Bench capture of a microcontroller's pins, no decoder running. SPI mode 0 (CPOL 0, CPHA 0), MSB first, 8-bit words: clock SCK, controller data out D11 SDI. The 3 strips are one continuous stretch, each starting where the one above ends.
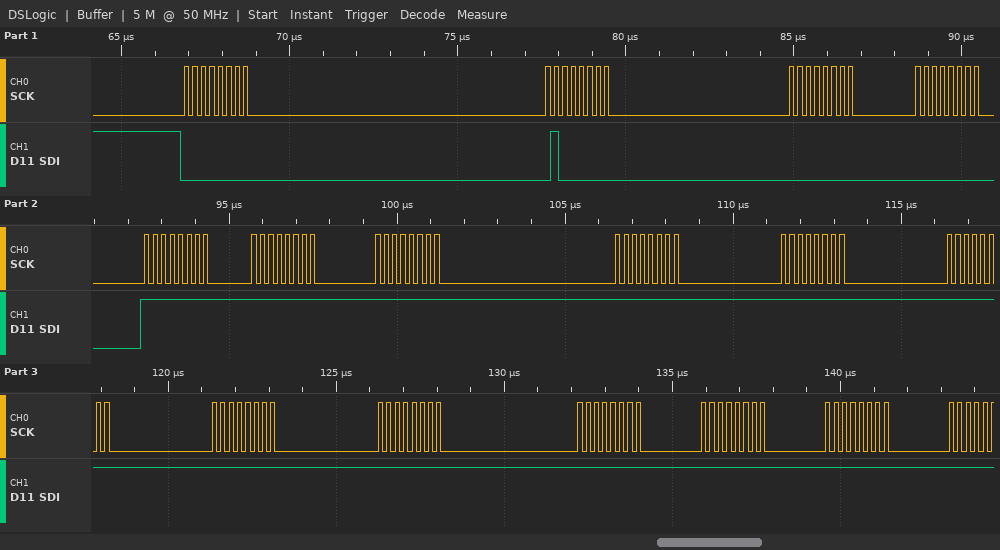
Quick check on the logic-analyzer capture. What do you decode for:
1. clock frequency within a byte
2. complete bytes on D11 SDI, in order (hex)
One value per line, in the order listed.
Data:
4 MHz
00 40 00 00 FF FF FF FF FF FF FF FF FF FF FF
